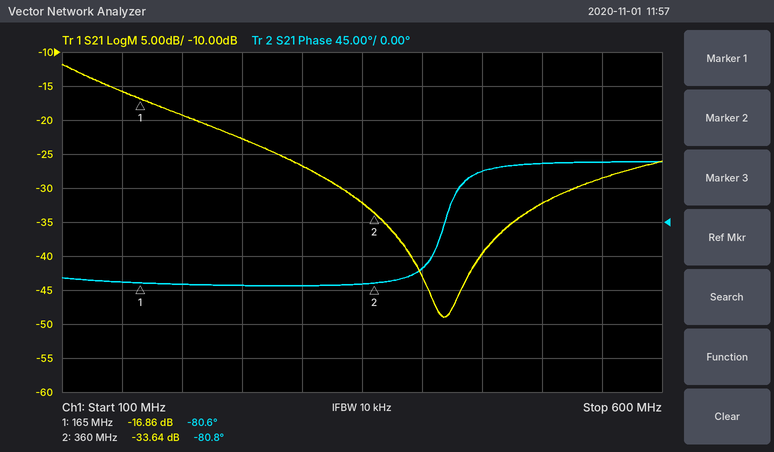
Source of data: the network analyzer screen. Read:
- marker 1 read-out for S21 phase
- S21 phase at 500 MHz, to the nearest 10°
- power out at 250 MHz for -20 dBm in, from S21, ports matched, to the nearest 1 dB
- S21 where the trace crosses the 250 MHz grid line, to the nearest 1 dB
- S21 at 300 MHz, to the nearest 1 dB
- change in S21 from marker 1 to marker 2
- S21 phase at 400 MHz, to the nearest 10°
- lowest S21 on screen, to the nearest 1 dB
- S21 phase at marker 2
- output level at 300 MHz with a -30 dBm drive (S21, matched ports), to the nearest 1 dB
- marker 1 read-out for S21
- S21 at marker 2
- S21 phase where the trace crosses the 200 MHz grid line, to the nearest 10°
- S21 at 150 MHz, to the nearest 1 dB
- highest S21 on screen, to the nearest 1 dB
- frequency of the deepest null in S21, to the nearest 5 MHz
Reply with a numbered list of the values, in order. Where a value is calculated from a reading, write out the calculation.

1. -80.6°
2. 80°
3. -20 dBm + (-23 dB) = -43 dBm
4. -23 dB
5. -27 dB
6. -33.64 − (-16.86) = -16.78 dB
7. -60°
8. -49 dB
9. -80.8°
10. -30 dBm + (-27 dB) = -57 dBm
11. -16.86 dB
12. -33.64 dB
13. -80°
14. -16 dB
15. -12 dB
16. 420 MHz
